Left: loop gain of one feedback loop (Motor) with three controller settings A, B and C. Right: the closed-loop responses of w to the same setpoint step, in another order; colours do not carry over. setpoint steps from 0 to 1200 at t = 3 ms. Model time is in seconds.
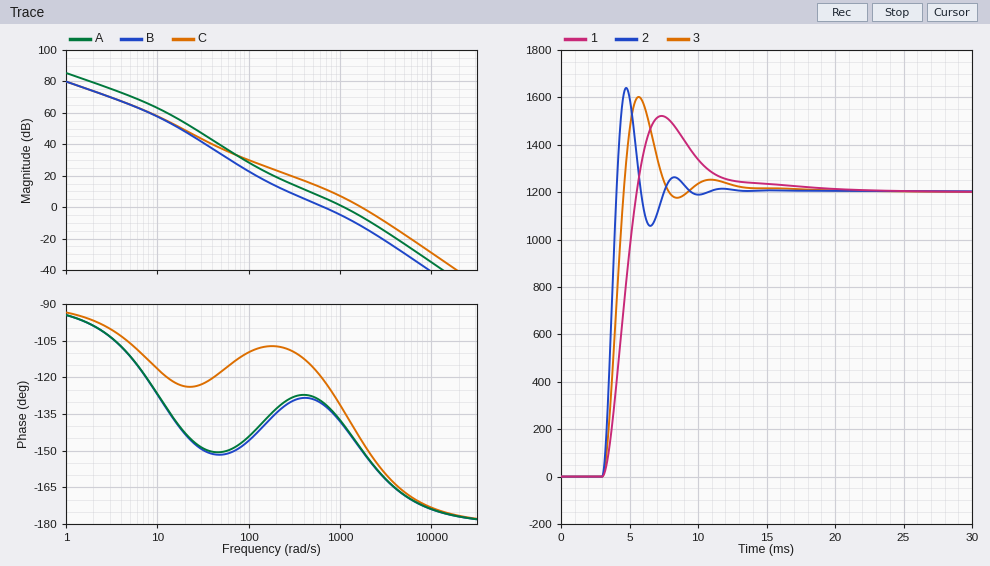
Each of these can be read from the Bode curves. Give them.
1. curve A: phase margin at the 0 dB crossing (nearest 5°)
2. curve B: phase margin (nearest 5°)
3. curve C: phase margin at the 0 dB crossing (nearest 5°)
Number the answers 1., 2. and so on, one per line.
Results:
1. 40°
2. 50°
3. 35°
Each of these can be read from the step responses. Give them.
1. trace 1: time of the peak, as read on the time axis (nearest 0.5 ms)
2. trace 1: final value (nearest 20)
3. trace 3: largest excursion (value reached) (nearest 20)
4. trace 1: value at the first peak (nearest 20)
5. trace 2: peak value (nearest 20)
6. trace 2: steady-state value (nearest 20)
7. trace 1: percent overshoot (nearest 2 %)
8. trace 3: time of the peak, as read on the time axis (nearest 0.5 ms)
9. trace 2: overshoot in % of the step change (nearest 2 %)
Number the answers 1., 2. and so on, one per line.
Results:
1. 7.5 ms
2. 1200
3. 1600
4. 1520
5. 1640
6. 1200
7. 26 %
8. 5.5 ms
9. 36 %
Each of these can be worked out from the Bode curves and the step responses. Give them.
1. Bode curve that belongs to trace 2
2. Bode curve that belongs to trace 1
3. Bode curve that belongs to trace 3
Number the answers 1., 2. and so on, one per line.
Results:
1. C
2. B
3. A
